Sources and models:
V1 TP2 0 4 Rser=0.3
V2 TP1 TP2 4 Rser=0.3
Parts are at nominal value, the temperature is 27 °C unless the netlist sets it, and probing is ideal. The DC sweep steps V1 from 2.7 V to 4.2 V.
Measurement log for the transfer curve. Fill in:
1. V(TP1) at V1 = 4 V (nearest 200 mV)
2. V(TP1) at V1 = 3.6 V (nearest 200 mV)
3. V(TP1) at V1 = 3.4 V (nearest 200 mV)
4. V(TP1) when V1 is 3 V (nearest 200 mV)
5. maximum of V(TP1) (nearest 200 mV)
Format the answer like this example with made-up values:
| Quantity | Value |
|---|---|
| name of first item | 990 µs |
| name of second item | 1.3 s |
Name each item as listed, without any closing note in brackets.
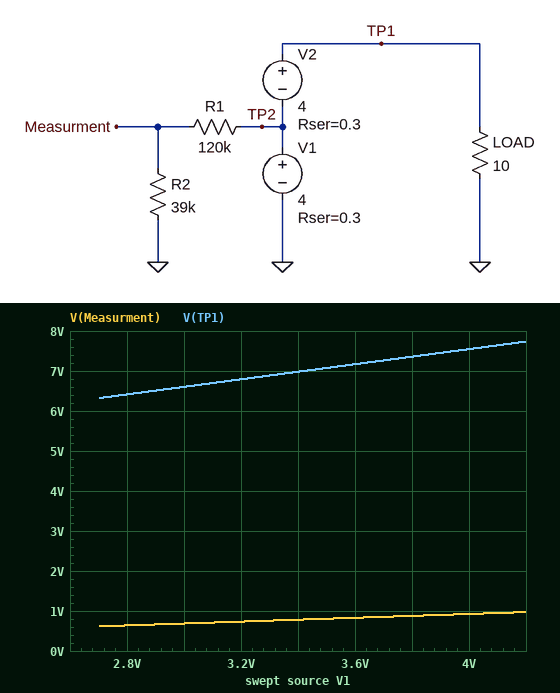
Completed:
| Quantity | Value |
|---|---|
| V(TP1) at V1 = 4 V | 7.6 V |
| V(TP1) at V1 = 3.6 V | 7.2 V |
| V(TP1) at V1 = 3.4 V | 7.0 V |
| V(TP1) when V1 is 3 V | 6.6 V |
| maximum of V(TP1) | 7.8 V |
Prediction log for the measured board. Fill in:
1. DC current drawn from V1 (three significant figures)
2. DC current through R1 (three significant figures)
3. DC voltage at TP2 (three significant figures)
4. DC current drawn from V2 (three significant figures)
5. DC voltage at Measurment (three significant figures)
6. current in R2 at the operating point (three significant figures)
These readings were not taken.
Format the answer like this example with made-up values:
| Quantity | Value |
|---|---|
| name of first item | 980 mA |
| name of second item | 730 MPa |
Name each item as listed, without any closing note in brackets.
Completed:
| Quantity | Value |
|---|---|
| DC current drawn from V1 | 755 mA |
| DC current through R1 | 23.7 µA |
| DC voltage at TP2 | 3.77 V |
| DC current drawn from V2 | 755 mA |
| DC voltage at Measurment | 926 mV |
| current in R2 at the operating point | 23.7 µA |
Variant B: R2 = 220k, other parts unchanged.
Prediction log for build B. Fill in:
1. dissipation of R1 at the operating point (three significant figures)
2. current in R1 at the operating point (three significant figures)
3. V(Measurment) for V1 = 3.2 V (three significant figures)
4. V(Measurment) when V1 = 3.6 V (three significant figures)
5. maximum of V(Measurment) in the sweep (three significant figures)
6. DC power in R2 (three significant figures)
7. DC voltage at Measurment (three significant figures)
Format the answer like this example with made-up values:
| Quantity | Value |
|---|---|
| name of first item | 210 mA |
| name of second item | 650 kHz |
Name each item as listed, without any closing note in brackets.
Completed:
| Quantity | Value |
|---|---|
| dissipation of R1 at the operating point | 14.8 µW |
| current in R1 at the operating point | 11.1 µA |
| V(Measurment) for V1 = 3.2 V | 1.94 V |
| V(Measurment) when V1 = 3.6 V | 2.19 V |
| maximum of V(Measurment) in the sweep | 2.57 V |
| DC power in R2 | 27.1 µW |
| DC voltage at Measurment | 2.44 V |
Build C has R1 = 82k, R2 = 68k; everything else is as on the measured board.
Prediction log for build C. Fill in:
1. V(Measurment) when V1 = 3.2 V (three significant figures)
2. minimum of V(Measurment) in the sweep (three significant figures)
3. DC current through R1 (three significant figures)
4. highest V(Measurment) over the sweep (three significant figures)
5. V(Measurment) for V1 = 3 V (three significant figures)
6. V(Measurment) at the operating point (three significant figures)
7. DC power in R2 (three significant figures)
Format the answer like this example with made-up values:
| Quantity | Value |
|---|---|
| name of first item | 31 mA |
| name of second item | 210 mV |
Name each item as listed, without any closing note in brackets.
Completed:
| Quantity | Value |
|---|---|
| V(Measurment) when V1 = 3.2 V | 1.36 V |
| minimum of V(Measurment) in the sweep | 1.14 V |
| DC current through R1 | 25.2 µA |
| highest V(Measurment) over the sweep | 1.80 V |
| V(Measurment) for V1 = 3 V | 1.27 V |
| V(Measurment) at the operating point | 1.71 V |
| DC power in R2 | 43.0 µW |
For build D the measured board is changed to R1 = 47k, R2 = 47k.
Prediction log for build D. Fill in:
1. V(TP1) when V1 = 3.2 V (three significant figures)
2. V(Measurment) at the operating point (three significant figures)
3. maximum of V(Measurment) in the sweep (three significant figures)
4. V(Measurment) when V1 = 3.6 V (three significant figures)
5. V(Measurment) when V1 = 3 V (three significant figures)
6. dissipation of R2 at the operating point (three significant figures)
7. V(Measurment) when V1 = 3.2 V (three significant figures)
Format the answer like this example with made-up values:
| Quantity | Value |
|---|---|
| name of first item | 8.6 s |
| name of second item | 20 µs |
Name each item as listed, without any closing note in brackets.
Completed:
| Quantity | Value |
|---|---|
| V(TP1) when V1 = 3.2 V | 6.79 V |
| V(Measurment) at the operating point | 1.89 V |
| maximum of V(Measurment) in the sweep | 1.98 V |
| V(Measurment) when V1 = 3.6 V | 1.69 V |
| V(Measurment) when V1 = 3 V | 1.40 V |
| dissipation of R2 at the operating point | 75.7 µW |
| V(Measurment) when V1 = 3.2 V | 1.50 V |
